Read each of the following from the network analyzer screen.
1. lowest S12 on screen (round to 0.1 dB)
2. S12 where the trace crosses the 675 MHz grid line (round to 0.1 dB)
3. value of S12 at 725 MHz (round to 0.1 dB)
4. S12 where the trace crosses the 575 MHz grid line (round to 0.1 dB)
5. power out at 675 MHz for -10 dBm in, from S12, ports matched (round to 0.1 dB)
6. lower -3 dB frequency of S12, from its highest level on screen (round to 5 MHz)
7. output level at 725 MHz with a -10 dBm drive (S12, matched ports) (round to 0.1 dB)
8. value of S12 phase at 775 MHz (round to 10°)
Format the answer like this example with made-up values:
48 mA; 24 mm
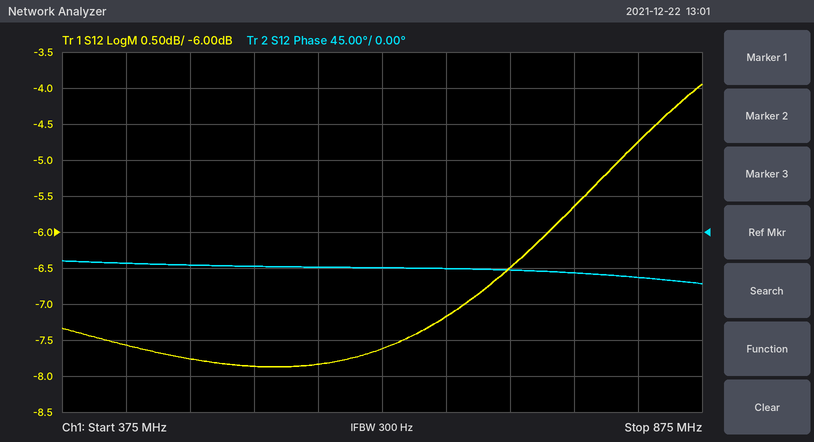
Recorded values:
-7.9 dB; -7.2 dB; -6.5 dB; -7.8 dB; -17.2 dBm; 695 MHz; -16.5 dBm; -50°
